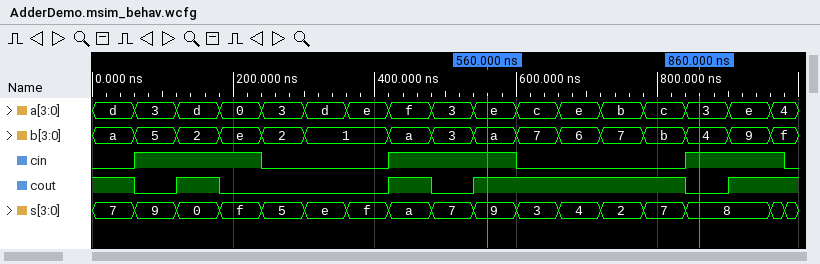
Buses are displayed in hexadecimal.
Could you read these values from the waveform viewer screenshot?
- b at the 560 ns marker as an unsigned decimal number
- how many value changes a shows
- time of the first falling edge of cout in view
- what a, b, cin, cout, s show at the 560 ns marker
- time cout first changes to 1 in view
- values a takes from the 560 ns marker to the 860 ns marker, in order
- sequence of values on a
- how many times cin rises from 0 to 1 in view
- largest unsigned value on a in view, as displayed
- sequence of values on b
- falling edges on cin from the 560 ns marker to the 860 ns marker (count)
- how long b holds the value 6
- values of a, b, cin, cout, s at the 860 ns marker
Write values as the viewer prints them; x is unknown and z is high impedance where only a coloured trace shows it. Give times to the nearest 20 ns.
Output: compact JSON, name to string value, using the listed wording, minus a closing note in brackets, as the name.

{"b at the 560 ns marker as an unsigned decimal number": "10", "how many value changes a shows": "16", "time of the first falling edge of cout in view": "60 ns", "what a, b, cin, cout, s show at the 560 ns marker": "a=e, b=a, cin=1, cout=1, s=9", "time cout first changes to 1 in view": "120 ns", "values a takes from the 560 ns marker to the 860 ns marker, in order": "e, c, e, b, c, 3", "sequence of values on a": "d, 3, d, 0, 3, d, e, f, 3, e, c, e, b, c, 3, e, 4", "how many times cin rises from 0 to 1 in view": "3", "largest unsigned value on a in view, as displayed": "f", "sequence of values on b": "a, 5, 2, e, 2, 1, a, 3, a, 7, 6, 7, b, 4, 9, f", "falling edges on cin from the 560 ns marker to the 860 ns marker": "1", "how long b holds the value 6": "60 ns", "values of a, b, cin, cout, s at the 860 ns marker": "a=3, b=4, cin=1, cout=0, s=8"}
